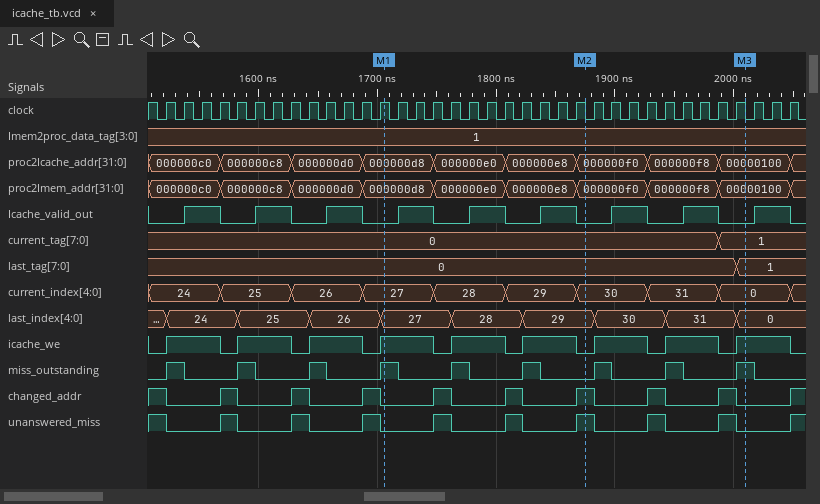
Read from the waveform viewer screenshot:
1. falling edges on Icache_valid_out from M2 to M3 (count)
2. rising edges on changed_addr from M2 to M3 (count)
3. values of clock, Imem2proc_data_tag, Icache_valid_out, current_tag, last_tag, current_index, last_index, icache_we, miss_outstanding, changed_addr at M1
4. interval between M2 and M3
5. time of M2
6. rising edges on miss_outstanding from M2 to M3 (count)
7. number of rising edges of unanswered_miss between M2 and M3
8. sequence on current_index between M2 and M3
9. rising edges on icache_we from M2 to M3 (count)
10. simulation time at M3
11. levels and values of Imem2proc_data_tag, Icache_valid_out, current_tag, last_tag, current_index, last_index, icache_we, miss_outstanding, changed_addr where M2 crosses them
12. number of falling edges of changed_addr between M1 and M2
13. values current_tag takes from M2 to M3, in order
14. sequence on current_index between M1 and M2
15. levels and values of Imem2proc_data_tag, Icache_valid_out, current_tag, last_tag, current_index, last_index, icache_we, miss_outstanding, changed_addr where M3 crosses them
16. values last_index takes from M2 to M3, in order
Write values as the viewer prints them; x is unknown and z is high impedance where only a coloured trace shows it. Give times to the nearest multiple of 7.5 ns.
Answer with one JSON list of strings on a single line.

["2", "2", "clock=1, Imem2proc_data_tag=1, Icache_valid_out=0, current_tag=0, last_tag=0, current_index=27, last_index=27, icache_we=1, miss_outstanding=1, changed_addr=0", "135 ns", "1875 ns", "3", "2", "30, 31, 0", "3", "2010 ns", "Imem2proc_data_tag=1, Icache_valid_out=0, current_tag=0, last_tag=0, current_index=30, last_index=29, icache_we=0, miss_outstanding=0, changed_addr=1", "2", "0, 1", "27, 28, 29, 30", "Imem2proc_data_tag=1, Icache_valid_out=0, current_tag=1, last_tag=1, current_index=0, last_index=0, icache_we=1, miss_outstanding=1, changed_addr=0", "29, 30, 31, 0"]
